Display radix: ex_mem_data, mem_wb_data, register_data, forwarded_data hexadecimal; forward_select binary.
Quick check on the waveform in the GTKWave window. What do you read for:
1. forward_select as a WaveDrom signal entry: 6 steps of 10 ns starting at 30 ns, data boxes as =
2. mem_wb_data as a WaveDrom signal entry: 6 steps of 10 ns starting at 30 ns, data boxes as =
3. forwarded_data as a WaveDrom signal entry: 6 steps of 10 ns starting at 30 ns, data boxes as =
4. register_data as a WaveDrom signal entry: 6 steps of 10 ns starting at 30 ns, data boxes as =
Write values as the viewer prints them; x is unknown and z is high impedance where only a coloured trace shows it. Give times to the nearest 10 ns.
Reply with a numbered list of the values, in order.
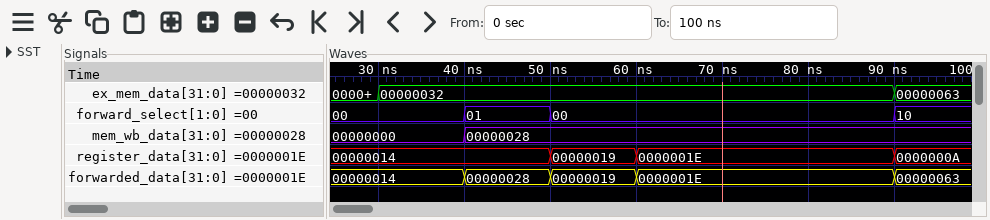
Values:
1. {name: 'forward_select', wave: '===...', data: '00 01 00'}
2. {name: 'mem_wb_data', wave: '==....', data: '00000000 00000028'}
3. {name: 'forwarded_data', wave: '====..', data: '00000014 00000028 00000019 0000001E'}
4. {name: 'register_data', wave: '=.==..', data: '00000014 00000019 0000001E'}
